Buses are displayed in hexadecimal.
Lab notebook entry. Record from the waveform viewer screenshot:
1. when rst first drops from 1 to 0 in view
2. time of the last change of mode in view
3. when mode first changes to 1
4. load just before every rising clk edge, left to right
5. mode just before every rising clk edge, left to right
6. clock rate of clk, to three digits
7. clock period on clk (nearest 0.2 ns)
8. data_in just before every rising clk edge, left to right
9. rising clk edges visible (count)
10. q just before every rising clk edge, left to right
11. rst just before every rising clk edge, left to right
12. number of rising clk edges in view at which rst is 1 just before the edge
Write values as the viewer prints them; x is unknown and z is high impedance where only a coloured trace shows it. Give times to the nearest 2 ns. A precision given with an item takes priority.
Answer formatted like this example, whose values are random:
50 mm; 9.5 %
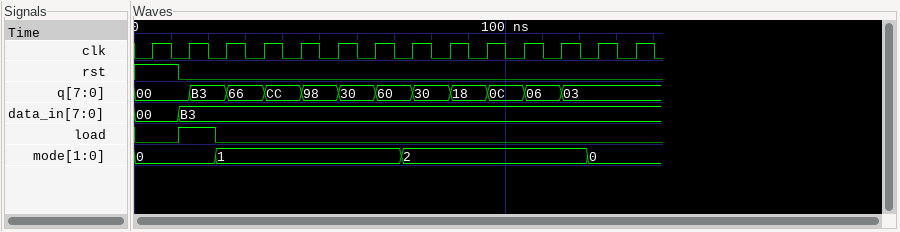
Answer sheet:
12 ns; 122 ns; 22 ns; 0 1 0 0 0 0 0 0 0 0 0 0 0 0; 0, 0, 1, 1, 1, 1, 1, 2, 2, 2, 2, 2, 0, 0; 100 MHz; 10 ns; 00, B3, B3, B3, B3, B3, B3, B3, B3, B3, B3, B3, B3, B3; 14; 00, 00, B3, 66, CC, 98, 30, 60, 30, 18, 0C, 06, 03, 03; 1 0 0 0 0 0 0 0 0 0 0 0 0 0; 1
